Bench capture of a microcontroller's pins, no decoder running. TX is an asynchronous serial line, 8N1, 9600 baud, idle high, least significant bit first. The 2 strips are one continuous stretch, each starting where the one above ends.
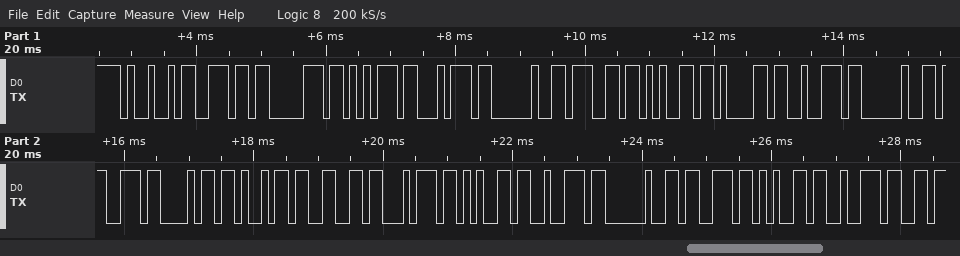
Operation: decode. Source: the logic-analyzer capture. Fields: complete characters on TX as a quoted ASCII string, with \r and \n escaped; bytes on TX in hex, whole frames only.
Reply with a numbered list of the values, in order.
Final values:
1. "Input gear shifter ser"
2. 49 6E 70 75 74 20 67 65 61 72 20 73 68 69 66 74 65 72 20 73 65 72
